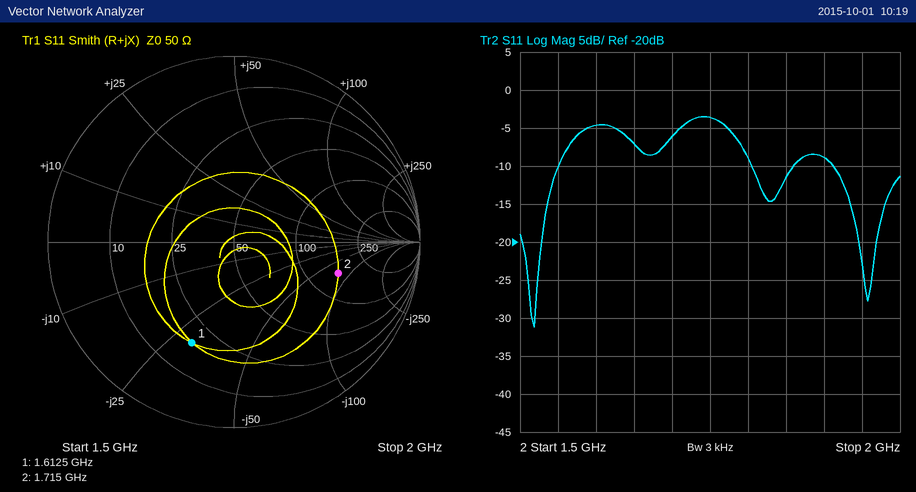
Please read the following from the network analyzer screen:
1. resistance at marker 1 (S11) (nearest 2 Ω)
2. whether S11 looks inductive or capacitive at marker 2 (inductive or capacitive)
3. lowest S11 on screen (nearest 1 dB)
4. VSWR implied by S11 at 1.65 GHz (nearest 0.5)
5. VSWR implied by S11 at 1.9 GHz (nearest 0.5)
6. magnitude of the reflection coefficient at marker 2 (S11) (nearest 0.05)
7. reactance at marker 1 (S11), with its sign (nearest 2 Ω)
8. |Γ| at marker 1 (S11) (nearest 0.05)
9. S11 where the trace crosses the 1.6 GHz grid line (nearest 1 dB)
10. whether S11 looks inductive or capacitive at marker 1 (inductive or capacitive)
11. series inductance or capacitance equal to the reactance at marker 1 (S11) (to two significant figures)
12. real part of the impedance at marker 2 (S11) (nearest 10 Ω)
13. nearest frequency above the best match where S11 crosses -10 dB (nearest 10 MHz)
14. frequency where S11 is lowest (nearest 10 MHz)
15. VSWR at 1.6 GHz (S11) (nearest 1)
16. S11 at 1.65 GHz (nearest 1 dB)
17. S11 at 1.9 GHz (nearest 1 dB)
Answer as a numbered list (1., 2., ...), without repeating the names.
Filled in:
1. 18 Ω
2. capacitive
3. -31 dB
4. 2.5
5. 2.0
6. 0.60
7. -30 Ω
8. 0.60
9. -5 dB
10. capacitive
11. 3.3 pF
12. 150 Ω
13. 1.55 GHz
14. 1.52 GHz
15. 4
16. -7 dB
17. -9 dB
